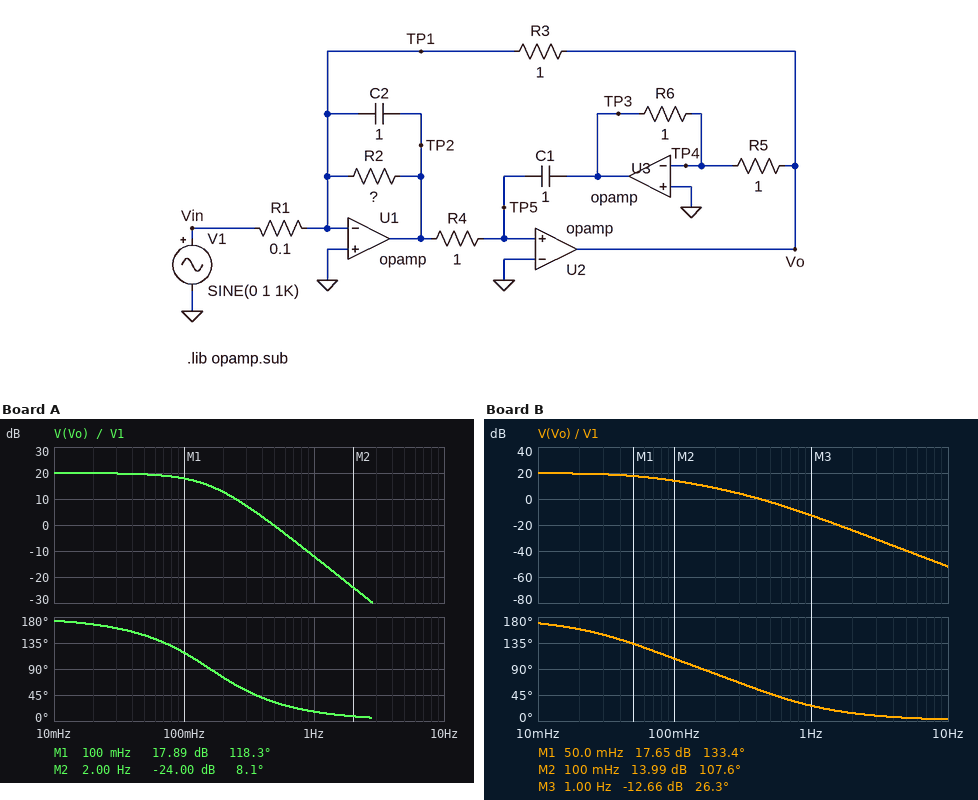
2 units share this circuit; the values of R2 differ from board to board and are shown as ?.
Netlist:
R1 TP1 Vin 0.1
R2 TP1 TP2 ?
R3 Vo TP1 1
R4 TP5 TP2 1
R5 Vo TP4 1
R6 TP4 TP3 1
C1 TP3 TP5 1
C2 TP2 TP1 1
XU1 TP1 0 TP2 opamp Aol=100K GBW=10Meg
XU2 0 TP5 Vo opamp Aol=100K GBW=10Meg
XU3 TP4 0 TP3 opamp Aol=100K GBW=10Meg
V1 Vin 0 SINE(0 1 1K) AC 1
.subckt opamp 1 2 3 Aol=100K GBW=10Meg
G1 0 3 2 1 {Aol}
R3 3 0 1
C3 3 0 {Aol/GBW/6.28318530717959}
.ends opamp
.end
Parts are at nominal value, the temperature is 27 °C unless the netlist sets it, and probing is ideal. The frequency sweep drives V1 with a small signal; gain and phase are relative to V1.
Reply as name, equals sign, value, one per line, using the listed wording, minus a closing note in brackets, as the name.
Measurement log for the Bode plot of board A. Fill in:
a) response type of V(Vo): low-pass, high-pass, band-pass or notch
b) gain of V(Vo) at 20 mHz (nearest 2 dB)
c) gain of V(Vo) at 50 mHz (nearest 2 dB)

response type of V(Vo): low-pass, high-pass, band-pass or notch = low-pass
gain of V(Vo) at 20 mHz = 20 dB
gain of V(Vo) at 50 mHz = 20 dB
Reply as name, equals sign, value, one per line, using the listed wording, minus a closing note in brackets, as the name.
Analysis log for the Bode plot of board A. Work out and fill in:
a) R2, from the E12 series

R2, from the E12 series = 0.56 Ω
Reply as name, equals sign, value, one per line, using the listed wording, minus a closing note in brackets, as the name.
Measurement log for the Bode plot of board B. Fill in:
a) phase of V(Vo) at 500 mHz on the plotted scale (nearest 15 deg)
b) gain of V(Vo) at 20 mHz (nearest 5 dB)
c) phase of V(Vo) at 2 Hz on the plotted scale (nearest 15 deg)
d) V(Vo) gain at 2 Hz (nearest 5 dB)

phase of V(Vo) at 500 mHz on the plotted scale = 45 deg
gain of V(Vo) at 20 mHz = 20 dB
phase of V(Vo) at 2 Hz on the plotted scale = 15 deg
V(Vo) gain at 2 Hz = -25 dB
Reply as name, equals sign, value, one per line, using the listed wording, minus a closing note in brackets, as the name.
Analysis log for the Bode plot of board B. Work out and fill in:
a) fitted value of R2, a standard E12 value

fitted value of R2, a standard E12 value = 0.33 Ω
